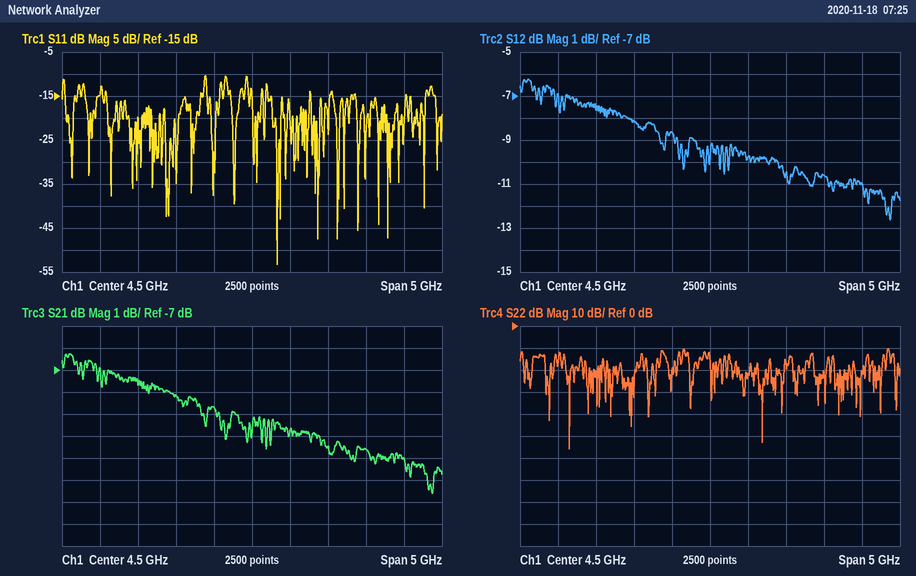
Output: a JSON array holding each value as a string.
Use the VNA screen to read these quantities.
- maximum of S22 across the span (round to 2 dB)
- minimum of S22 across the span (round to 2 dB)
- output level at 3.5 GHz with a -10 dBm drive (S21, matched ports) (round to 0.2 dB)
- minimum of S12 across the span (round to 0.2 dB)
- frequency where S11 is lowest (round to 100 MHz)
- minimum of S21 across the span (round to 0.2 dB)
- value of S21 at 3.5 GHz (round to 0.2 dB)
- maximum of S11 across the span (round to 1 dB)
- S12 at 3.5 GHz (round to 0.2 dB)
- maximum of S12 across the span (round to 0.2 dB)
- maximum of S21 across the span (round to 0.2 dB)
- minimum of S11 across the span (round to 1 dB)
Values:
["-10 dB", "-56 dB", "-18.2 dBm", "-12.6 dB", "4.8 GHz", "-12.6 dB", "-8.2 dB", "-10 dB", "-8.2 dB", "-6.2 dB", "-6.2 dB", "-53 dB"]
